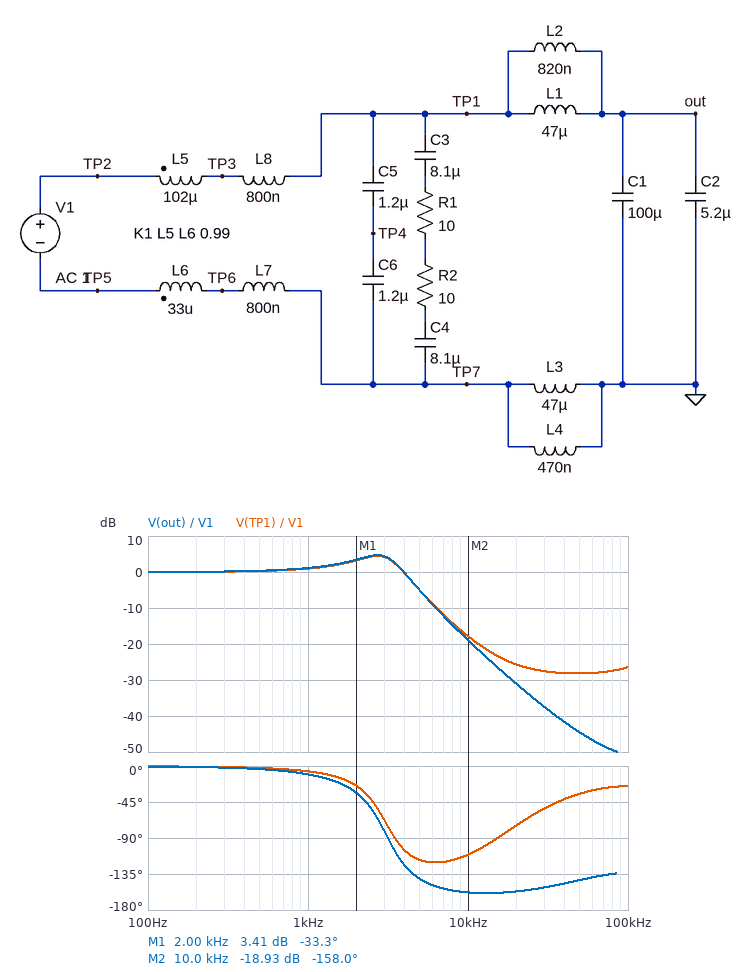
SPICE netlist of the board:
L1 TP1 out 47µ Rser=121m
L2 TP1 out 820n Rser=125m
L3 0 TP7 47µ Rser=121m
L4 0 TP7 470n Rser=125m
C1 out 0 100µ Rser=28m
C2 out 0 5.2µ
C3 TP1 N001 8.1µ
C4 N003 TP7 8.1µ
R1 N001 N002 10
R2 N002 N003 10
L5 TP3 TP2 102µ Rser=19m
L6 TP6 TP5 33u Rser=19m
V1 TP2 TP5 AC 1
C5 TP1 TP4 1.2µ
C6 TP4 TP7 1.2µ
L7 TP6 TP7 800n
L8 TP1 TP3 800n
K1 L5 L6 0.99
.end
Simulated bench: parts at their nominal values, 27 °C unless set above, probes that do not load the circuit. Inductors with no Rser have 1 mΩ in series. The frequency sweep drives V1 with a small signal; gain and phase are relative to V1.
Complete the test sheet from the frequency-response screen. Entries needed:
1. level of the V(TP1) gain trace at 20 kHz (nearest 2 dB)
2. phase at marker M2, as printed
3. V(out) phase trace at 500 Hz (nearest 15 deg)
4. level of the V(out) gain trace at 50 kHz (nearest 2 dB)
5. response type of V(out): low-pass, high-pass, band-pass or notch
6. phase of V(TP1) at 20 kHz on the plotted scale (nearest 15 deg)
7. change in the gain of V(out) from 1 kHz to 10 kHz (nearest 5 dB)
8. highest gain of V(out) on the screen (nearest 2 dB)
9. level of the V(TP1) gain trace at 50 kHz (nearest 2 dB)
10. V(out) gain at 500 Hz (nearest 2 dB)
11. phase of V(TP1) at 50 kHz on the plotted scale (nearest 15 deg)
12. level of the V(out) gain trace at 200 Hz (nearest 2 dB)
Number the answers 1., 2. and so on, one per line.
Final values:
1. -26 dB
2. -158.0 deg
3. 0 deg
4. -44 dB
5. low-pass
6. -75 deg
7. -20 dB
8. 4 dB
9. -28 dB
10. 0 dB
11. -30 deg
12. 0 dB
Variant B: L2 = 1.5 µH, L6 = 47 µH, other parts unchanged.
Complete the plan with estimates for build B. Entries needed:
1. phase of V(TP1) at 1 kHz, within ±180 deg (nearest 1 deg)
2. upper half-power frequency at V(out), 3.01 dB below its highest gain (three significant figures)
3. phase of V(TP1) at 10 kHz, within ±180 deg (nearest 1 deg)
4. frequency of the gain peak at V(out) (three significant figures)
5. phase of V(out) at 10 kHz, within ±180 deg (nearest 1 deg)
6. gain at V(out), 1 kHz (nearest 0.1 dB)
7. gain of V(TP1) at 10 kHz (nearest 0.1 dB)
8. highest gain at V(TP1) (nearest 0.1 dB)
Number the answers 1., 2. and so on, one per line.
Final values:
1. -6 deg
2. 4.50 kHz
3. -92 deg
4. 3.10 kHz
5. -151 deg
6. 0.8 dB
7. -15.3 dB
8. 2.8 dB
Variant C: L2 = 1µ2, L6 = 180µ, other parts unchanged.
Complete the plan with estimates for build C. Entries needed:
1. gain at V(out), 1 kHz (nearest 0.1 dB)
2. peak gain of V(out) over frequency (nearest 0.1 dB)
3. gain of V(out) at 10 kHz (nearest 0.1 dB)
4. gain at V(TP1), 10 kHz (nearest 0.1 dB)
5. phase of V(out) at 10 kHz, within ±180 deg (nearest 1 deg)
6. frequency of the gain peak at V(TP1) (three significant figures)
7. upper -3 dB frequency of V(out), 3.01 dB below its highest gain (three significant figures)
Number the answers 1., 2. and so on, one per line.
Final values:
1. 0.9 dB
2. 3.5 dB
3. -16.1 dB
4. -15.7 dB
5. -153 deg
6. 3.01 kHz
7. 4.29 kHz
